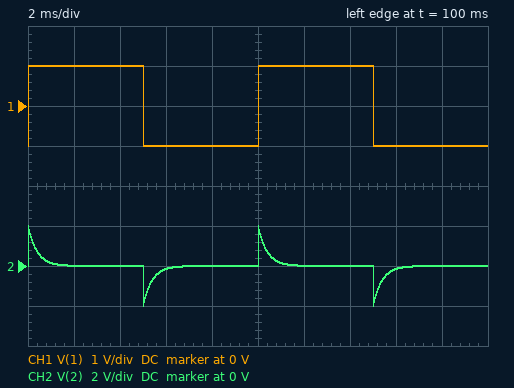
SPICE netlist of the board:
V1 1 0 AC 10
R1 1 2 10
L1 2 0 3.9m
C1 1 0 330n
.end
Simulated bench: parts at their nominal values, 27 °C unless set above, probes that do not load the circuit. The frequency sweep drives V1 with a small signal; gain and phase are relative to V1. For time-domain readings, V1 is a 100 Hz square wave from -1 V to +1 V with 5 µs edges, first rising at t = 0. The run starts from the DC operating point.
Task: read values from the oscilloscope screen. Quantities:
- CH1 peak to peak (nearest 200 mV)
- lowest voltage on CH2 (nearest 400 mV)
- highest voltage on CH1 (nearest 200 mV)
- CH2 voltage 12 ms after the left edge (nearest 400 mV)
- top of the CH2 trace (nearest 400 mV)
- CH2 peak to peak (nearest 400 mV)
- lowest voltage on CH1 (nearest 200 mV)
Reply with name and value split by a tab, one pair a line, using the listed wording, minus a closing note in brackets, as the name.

CH1 peak to peak	2.0 V
lowest voltage on CH2	-2.0 V
highest voltage on CH1	1.0 V
CH2 voltage 12 ms after the left edge	0 V
top of the CH2 trace	2.0 V
CH2 peak to peak	4.0 V
lowest voltage on CH1	-1.0 V
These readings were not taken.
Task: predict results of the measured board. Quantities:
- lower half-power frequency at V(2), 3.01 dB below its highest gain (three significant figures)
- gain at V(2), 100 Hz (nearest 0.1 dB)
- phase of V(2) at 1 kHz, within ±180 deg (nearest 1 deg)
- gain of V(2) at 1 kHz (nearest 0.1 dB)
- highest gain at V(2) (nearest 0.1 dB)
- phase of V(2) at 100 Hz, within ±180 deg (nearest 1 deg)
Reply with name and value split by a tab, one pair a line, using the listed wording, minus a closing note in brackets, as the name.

lower half-power frequency at V(2), 3.01 dB below its highest gain	408 Hz
gain at V(2), 100 Hz	-12.5 dB
phase of V(2) at 1 kHz, within ±180 deg	22 deg
gain of V(2) at 1 kHz	-0.7 dB
highest gain at V(2)	0 dB
phase of V(2) at 100 Hz, within ±180 deg	76 deg
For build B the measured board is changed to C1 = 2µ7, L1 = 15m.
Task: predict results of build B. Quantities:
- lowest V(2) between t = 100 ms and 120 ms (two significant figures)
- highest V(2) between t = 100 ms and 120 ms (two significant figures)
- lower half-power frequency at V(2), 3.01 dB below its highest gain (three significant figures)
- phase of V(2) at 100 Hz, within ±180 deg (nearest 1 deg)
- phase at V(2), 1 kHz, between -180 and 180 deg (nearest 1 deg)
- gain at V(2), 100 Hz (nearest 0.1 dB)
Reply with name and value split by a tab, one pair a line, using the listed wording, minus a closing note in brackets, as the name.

lowest V(2) between t = 100 ms and 120 ms	-1.9 V
highest V(2) between t = 100 ms and 120 ms	1.9 V
lower half-power frequency at V(2), 3.01 dB below its highest gain	106 Hz
phase of V(2) at 100 Hz, within ±180 deg	47 deg
phase at V(2), 1 kHz, between -180 and 180 deg	6 deg
gain at V(2), 100 Hz	-3.3 dB
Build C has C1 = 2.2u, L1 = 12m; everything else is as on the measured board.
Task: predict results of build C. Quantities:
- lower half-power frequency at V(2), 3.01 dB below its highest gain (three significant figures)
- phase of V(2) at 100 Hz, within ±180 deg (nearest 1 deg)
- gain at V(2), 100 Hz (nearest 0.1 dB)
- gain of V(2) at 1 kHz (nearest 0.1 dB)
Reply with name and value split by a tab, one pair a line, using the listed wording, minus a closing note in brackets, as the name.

lower half-power frequency at V(2), 3.01 dB below its highest gain	133 Hz
phase of V(2) at 100 Hz, within ±180 deg	53 deg
gain at V(2), 100 Hz	-4.4 dB
gain of V(2) at 1 kHz	-0.1 dB
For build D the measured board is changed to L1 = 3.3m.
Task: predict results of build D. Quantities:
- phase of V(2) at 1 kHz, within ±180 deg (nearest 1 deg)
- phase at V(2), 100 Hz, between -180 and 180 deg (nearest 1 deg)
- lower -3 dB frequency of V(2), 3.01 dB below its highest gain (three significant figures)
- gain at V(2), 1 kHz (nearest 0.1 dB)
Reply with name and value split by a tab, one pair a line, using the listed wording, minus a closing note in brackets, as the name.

phase of V(2) at 1 kHz, within ±180 deg	26 deg
phase at V(2), 100 Hz, between -180 and 180 deg	78 deg
lower -3 dB frequency of V(2), 3.01 dB below its highest gain	482 Hz
gain at V(2), 1 kHz	-0.9 dB
